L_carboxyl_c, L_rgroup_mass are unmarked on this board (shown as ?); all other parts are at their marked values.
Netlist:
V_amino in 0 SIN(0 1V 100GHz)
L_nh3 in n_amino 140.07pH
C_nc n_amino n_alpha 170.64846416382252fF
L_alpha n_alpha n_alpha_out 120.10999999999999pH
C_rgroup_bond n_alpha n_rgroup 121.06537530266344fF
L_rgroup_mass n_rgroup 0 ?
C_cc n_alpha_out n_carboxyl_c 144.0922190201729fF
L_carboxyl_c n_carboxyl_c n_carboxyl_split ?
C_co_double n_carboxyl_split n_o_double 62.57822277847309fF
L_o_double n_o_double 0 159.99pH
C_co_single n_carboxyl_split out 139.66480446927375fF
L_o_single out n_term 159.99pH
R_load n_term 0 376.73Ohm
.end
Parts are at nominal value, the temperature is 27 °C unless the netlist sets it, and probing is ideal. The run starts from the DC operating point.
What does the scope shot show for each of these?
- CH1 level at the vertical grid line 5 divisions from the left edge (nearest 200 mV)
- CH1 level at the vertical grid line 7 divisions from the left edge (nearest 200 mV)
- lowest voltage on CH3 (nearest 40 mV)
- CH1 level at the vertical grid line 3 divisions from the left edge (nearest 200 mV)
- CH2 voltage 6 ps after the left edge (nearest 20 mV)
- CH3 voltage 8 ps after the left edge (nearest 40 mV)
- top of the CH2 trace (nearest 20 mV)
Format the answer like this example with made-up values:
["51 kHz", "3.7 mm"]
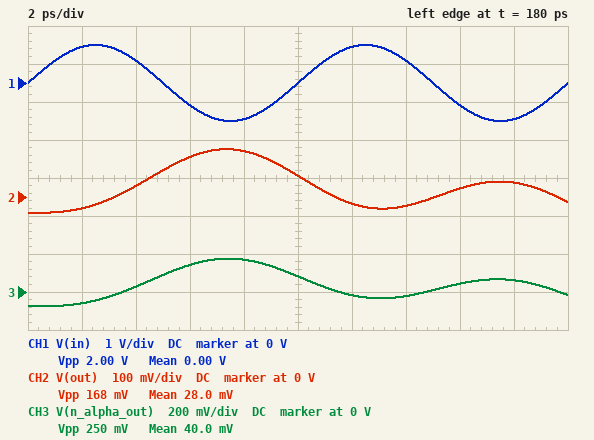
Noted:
["0 V", "600 mV", "-80 mV", "-600 mV", "100 mV", "160 mV", "120 mV"]
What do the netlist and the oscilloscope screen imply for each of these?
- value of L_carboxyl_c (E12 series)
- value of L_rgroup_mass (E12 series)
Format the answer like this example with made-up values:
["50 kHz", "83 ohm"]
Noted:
["68 pH", "8.2 pH"]
